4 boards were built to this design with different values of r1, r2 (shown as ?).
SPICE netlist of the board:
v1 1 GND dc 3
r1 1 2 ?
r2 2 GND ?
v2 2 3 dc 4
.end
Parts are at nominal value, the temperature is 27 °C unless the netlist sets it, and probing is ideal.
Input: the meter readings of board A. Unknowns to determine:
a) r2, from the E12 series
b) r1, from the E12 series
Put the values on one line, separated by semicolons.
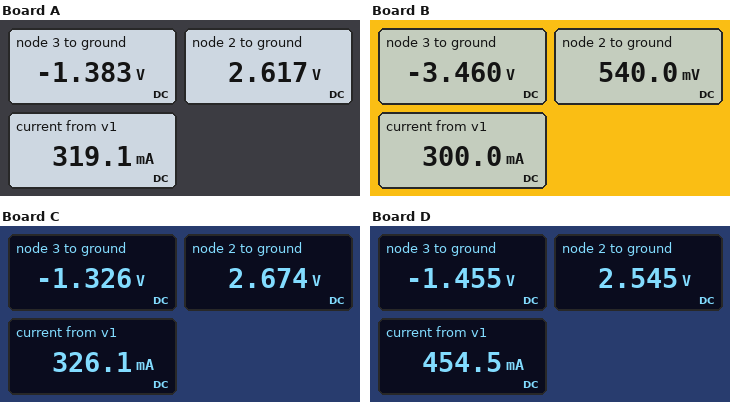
8.2 Ω; 1.2 Ω
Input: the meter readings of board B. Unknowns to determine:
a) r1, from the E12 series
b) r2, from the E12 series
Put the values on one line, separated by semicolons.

8.2 Ω; 1.8 Ω
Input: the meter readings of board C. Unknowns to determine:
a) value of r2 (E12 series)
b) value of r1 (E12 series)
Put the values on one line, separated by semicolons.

8.2 Ω; 1 Ω
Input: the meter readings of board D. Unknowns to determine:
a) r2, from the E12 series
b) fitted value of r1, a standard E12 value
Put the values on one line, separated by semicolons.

5.6 Ω; 1 Ω
